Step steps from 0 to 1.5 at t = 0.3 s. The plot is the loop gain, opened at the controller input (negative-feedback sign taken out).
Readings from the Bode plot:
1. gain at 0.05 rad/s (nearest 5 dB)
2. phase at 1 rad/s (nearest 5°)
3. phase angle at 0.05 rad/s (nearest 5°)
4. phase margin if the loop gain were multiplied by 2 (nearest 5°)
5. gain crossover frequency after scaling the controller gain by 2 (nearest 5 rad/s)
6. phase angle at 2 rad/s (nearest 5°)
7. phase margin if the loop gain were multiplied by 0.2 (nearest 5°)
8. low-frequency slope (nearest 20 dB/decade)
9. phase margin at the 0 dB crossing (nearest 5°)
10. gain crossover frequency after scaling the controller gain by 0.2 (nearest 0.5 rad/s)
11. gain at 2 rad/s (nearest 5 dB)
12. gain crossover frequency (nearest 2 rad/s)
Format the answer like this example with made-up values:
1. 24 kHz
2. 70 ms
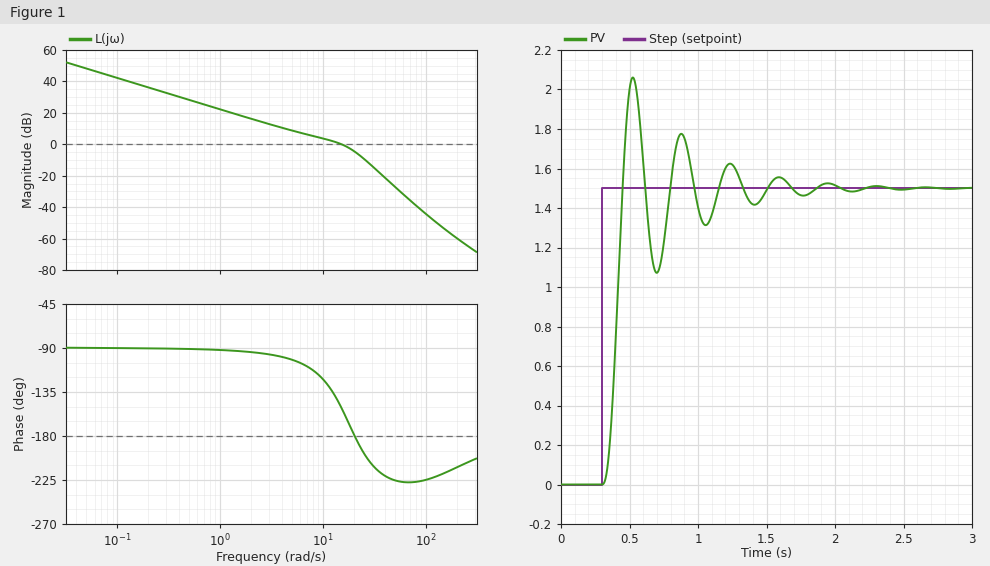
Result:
1. 50 dB
2. -90°
3. -90°
4. -5°
5. 20 rad/s
6. -95°
7. 85°
8. -20 dB/decade
9. 30°
10. 2.5 rad/s
11. 15 dB
12. 16 rad/s
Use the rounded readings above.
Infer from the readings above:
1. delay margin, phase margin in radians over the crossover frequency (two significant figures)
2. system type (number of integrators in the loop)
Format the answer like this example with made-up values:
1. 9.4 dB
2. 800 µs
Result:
1. 0.033 s
2. 1
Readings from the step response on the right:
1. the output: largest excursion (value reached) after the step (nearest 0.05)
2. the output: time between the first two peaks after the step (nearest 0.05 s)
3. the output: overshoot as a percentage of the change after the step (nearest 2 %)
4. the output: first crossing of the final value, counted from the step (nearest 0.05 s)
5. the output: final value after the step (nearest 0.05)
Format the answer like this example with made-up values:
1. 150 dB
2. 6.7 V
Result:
1. 2.05
2. 0.35 s
3. 38 %
4. 0.15 s
5. 1.50
